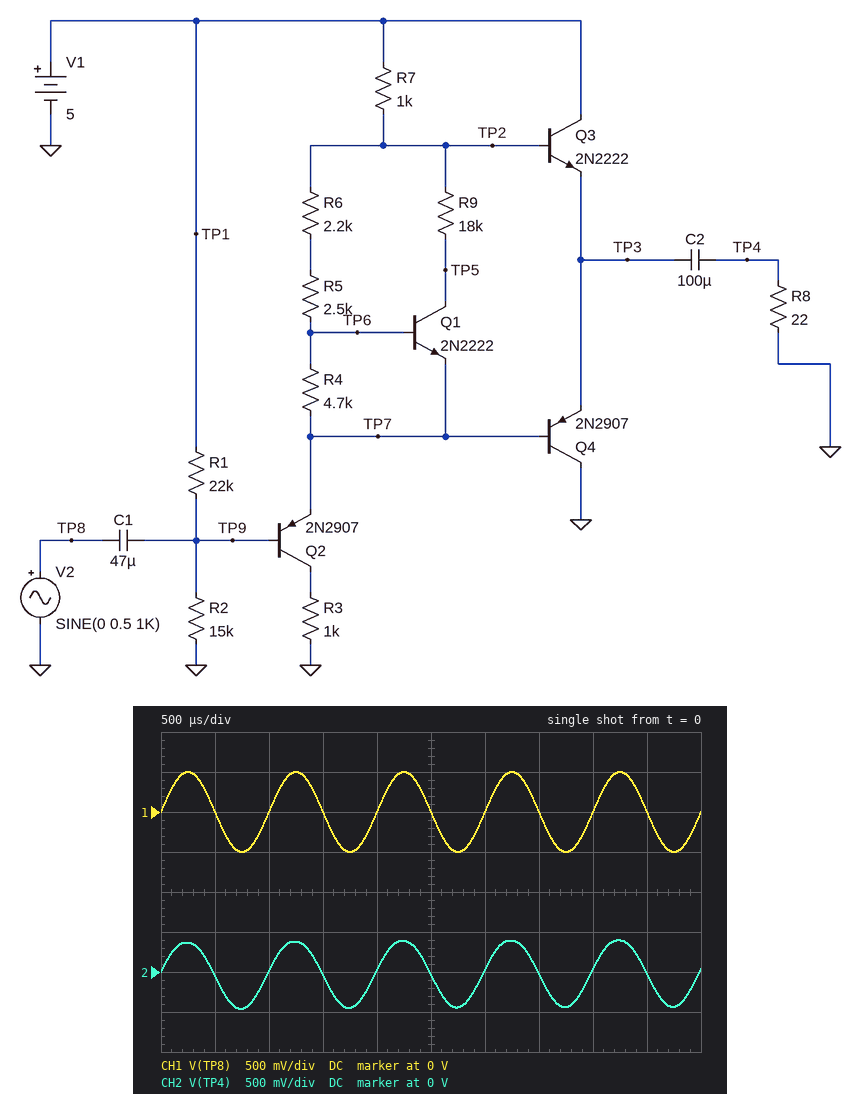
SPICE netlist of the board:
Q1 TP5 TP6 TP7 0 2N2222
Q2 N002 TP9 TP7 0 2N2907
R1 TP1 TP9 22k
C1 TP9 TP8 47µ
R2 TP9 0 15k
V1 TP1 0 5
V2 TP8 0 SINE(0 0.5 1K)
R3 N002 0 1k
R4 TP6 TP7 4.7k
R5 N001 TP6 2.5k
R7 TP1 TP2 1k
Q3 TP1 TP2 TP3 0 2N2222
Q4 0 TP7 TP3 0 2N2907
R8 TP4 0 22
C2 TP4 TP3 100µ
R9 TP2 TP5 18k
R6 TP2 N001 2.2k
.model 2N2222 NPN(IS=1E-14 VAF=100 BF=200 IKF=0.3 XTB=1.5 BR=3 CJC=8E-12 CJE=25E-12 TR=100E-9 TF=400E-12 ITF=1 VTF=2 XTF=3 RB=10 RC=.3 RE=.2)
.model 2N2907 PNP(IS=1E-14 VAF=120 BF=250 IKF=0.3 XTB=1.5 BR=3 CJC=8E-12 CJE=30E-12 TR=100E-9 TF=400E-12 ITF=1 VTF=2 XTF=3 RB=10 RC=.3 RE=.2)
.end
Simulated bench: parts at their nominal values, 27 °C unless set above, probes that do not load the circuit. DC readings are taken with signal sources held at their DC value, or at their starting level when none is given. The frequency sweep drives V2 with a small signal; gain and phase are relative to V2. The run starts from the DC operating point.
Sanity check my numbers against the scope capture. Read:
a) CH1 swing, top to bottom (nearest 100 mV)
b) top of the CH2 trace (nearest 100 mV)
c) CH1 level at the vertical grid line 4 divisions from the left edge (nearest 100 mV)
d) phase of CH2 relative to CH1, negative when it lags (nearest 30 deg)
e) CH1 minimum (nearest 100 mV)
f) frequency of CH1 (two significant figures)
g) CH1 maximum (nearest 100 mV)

1.0 V
400 mV
0 V
0 deg
-500 mV
1.0 kHz
500 mV
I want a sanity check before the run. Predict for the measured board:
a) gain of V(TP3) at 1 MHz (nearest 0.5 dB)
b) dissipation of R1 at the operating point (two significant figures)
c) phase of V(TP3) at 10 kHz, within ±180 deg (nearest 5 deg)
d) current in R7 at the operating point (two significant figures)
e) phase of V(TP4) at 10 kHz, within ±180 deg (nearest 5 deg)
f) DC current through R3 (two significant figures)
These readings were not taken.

-1.0 dB
400 µW
0 deg
730 µA
0 deg
630 µA
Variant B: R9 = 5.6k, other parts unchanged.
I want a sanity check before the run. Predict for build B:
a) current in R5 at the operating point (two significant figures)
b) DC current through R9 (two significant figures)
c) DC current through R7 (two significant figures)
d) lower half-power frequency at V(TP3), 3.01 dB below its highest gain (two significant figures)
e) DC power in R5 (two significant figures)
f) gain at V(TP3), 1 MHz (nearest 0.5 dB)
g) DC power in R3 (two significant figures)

190 µA
270 µA
760 µA
400 mHz
93 µW
-1.5 dB
480 µW
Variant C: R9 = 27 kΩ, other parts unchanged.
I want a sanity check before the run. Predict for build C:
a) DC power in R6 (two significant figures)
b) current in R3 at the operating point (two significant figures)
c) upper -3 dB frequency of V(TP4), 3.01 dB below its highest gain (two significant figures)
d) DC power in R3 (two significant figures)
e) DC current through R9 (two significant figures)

91 µW
620 µA
85 MHz
390 µW
58 µA
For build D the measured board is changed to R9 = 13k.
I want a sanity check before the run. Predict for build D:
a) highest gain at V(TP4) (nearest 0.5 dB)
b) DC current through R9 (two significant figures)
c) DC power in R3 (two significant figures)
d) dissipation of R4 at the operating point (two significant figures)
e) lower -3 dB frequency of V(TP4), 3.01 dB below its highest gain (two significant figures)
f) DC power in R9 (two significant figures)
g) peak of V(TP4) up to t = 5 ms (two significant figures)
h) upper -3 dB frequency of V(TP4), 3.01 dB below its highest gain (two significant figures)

-1.0 dB
120 µA
410 µW
85 µW
76 Hz
190 µW
390 mV
87 MHz
